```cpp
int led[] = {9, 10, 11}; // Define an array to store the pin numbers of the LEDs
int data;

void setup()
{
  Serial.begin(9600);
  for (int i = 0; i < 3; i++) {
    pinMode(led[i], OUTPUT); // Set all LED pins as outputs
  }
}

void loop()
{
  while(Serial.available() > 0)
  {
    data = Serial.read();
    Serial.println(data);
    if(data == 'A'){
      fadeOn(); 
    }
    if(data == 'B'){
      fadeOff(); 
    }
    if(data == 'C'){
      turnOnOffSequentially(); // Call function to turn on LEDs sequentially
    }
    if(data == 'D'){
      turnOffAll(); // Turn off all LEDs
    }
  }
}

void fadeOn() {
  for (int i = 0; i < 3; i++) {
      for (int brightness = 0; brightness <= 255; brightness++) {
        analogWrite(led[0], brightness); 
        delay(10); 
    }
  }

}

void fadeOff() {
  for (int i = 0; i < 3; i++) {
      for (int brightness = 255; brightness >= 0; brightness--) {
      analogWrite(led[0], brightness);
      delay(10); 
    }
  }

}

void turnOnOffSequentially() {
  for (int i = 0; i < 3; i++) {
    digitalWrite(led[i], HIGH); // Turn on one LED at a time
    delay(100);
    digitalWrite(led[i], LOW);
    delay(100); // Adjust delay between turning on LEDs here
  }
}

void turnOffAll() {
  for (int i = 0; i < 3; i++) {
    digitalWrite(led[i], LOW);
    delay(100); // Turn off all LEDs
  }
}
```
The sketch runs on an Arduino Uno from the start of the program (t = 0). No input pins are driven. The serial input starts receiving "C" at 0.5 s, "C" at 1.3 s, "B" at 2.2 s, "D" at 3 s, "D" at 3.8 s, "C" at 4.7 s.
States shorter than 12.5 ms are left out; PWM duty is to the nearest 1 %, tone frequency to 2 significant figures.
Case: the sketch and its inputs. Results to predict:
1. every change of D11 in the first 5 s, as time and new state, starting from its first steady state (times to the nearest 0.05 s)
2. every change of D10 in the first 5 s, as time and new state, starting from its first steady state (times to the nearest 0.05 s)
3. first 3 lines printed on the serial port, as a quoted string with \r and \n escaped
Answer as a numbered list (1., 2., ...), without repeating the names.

1. 0 s low; 0.9 s high; 1 s low; 1.7 s high; 1.8 s low
2. 0 s low; 0.7 s high; 0.8 s low; 1.5 s high; 1.6 s low
3. "67\r\n67\r\n66\r\n"
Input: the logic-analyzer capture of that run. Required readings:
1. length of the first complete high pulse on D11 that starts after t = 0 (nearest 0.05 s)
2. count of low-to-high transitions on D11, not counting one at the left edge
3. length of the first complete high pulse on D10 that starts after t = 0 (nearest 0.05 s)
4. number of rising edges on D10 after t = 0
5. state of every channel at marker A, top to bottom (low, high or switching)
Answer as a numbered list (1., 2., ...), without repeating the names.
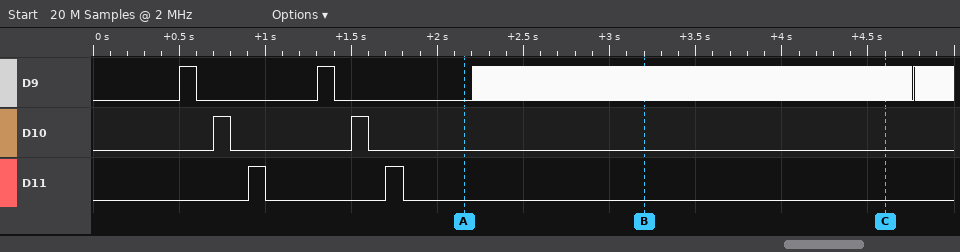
1. 0.10 s
2. 2
3. 0.10 s
4. 2
5. D9 low, D10 low, D11 low
